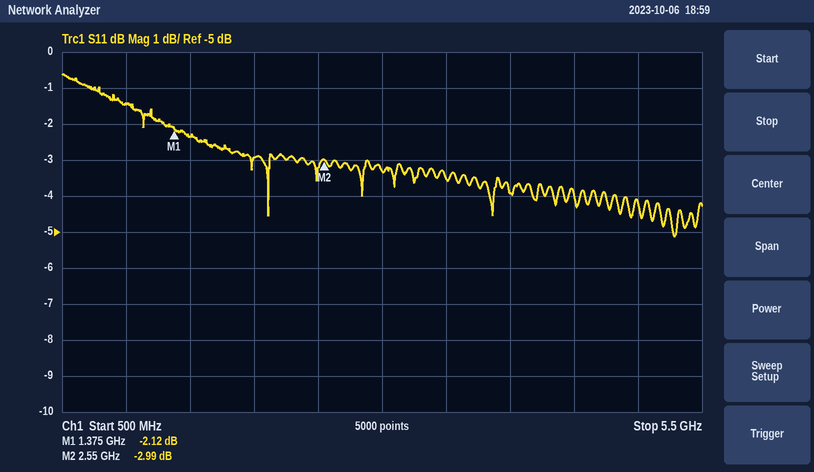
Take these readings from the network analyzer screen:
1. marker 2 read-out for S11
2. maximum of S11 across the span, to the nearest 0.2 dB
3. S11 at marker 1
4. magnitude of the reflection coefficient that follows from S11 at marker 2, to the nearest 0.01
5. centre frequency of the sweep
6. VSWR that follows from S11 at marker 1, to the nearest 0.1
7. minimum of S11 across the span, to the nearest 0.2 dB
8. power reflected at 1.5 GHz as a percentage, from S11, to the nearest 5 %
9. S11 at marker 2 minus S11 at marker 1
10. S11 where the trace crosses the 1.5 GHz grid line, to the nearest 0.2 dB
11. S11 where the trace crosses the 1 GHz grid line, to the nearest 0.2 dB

-2.99 dB
-0.6 dB
-2.12 dB
0.71
3 GHz
8.2
-5.2 dB
60 %
-0.87 dB
-2.4 dB
-1.4 dB
